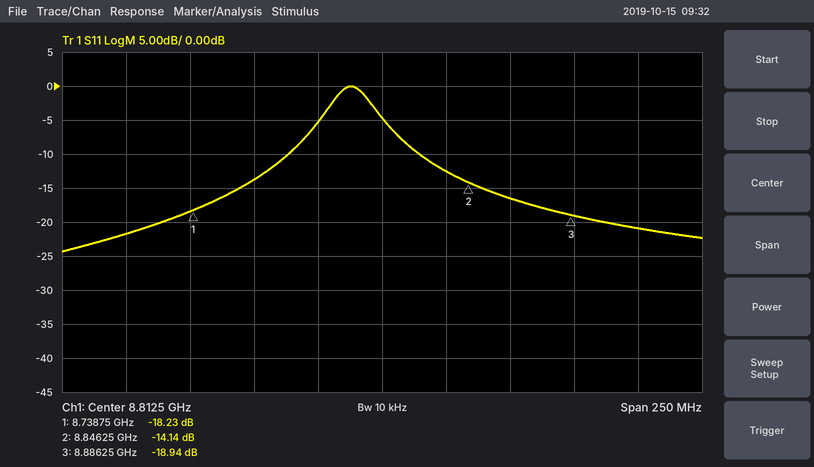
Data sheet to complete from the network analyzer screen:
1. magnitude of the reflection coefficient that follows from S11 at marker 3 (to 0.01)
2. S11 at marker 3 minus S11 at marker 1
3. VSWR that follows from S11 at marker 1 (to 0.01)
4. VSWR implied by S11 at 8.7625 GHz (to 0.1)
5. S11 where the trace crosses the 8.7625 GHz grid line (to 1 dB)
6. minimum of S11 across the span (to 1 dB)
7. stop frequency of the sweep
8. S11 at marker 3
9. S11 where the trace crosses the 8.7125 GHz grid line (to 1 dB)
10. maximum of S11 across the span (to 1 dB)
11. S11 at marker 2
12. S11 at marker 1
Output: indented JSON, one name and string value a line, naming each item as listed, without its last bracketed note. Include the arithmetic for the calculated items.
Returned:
{
  "magnitude of the reflection coefficient that follows from S11 at marker 3": "10^(-18.94/20) ≈ 0.11",
  "S11 at marker 3 minus S11 at marker 1": "-18.94 − (-18.23) = -0.71 dB",
  "VSWR that follows from S11 at marker 1": "(1 + 0.1226)/(1 − 0.1226) ≈ 1.28",
  "VSWR implied by S11 at 8.7625 GHz": "|Γ| = 10^(-14/20) = 0.1995; VSWR = (1 + 0.1995)/(1 − 0.1995) ≈ 1.5",
  "S11 where the trace crosses the 8.7625 GHz grid line": "-14 dB",
  "minimum of S11 across the span": "-24 dB",
  "stop frequency of the sweep": "8.9375 GHz",
  "S11 at marker 3": "-18.94 dB",
  "S11 where the trace crosses the 8.7125 GHz grid line": "-22 dB",
  "maximum of S11 across the span": "0 dB",
  "S11 at marker 2": "-14.14 dB",
  "S11 at marker 1": "-18.23 dB"
}
